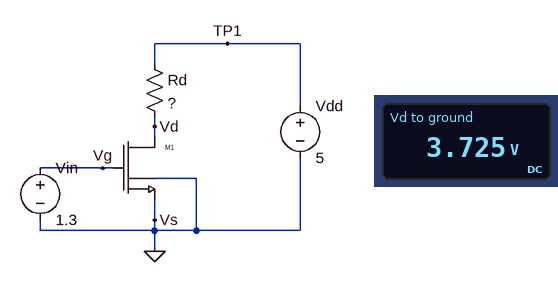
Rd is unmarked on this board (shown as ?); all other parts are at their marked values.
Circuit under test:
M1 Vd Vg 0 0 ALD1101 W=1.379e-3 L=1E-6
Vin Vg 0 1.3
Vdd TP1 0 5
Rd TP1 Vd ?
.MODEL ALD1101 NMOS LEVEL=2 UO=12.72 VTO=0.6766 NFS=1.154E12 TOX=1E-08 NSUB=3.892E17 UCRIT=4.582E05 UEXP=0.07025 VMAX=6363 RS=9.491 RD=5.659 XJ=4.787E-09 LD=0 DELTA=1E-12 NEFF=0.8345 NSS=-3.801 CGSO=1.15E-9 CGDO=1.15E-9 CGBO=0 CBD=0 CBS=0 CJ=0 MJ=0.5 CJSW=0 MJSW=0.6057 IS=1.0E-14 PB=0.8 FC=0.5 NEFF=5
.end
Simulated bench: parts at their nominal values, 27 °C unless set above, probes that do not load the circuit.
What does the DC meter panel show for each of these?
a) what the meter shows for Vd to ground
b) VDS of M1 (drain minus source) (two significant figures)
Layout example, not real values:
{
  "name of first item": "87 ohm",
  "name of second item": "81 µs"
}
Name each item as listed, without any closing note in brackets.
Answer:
{
  "what the meter shows for Vd to ground": "3.725 V",
  "VDS of M1 (drain minus source)": "3.7 V"
}
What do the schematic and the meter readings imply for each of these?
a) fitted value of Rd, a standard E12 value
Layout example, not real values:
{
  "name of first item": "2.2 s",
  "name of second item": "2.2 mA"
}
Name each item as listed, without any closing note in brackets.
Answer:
{
  "fitted value of Rd, a standard E12 value": "1.5 kΩ"
}
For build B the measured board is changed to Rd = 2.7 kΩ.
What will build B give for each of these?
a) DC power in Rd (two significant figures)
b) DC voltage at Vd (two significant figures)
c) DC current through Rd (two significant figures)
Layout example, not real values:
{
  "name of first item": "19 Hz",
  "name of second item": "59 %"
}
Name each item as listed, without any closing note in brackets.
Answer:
{
  "DC power in Rd": "1.9 mW",
  "DC voltage at Vd": "2.7 V",
  "DC current through Rd": "840 µA"
}
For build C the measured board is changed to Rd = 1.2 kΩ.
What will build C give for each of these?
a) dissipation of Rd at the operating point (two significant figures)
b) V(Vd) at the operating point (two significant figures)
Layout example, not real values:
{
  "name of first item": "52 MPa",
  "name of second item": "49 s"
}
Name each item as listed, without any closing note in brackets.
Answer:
{
  "dissipation of Rd at the operating point": "870 µW",
  "V(Vd) at the operating point": "4.0 V"
}
